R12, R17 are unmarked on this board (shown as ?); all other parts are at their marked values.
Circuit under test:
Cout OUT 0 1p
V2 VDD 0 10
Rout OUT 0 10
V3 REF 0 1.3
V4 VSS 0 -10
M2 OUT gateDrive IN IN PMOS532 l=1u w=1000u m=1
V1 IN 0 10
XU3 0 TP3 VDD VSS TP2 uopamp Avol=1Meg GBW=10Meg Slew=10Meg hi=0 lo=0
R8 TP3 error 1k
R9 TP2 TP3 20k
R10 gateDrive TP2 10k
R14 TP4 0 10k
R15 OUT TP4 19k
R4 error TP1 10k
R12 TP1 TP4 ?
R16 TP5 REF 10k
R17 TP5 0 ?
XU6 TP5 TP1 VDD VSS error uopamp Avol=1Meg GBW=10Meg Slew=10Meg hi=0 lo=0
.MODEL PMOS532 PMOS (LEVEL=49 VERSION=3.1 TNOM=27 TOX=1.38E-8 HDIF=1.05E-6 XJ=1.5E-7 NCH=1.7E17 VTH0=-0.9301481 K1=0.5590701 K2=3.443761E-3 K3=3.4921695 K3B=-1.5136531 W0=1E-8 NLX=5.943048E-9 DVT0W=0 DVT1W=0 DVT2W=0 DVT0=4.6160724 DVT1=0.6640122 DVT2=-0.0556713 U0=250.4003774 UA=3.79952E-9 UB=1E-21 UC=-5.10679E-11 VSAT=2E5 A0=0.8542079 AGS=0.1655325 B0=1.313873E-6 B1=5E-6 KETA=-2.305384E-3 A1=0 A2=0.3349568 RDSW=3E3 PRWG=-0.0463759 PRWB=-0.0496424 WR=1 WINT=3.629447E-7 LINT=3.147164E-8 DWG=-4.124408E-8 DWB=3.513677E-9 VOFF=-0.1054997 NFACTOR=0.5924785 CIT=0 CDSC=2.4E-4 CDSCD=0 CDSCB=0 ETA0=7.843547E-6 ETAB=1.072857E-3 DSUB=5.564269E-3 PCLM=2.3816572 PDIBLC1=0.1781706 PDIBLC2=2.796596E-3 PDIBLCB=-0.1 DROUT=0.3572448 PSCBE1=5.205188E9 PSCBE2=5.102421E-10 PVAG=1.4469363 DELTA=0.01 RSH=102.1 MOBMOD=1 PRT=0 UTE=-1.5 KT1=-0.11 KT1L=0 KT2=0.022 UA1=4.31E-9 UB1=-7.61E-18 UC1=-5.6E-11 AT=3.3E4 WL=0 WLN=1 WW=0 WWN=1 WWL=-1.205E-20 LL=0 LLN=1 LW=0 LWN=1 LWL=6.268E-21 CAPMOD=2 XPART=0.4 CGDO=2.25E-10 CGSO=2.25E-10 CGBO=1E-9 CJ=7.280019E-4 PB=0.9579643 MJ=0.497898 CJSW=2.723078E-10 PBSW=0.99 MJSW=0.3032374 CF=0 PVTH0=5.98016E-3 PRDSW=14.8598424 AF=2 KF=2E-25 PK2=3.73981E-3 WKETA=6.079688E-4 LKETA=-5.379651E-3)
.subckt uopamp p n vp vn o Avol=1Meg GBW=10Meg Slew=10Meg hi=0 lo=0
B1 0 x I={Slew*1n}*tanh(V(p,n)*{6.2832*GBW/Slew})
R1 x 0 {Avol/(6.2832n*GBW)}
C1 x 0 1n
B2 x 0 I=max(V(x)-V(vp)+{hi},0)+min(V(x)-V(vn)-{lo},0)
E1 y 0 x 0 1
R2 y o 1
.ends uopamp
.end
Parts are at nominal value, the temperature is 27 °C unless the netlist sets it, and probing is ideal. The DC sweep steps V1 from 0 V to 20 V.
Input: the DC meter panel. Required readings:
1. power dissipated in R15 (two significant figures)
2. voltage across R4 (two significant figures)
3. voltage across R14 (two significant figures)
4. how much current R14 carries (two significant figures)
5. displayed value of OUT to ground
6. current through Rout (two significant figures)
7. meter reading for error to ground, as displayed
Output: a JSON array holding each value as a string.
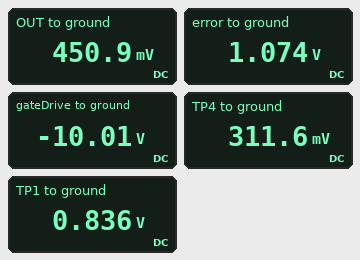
["1.0 µW", "240 mV", "310 mV", "31 µA", "450.9 mV", "45 mA", "1.074 V"]
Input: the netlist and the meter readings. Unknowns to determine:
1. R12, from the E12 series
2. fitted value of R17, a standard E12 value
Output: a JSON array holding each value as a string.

["22 kΩ", "18 kΩ"]
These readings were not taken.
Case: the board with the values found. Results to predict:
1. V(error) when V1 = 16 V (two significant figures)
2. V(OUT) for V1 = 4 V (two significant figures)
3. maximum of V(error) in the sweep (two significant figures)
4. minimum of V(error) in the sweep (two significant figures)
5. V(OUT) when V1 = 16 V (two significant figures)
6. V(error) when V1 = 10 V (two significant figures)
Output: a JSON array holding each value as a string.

["1.0 V", "180 mV", "1.1 V", "1.0 V", "720 mV", "1.1 V"]
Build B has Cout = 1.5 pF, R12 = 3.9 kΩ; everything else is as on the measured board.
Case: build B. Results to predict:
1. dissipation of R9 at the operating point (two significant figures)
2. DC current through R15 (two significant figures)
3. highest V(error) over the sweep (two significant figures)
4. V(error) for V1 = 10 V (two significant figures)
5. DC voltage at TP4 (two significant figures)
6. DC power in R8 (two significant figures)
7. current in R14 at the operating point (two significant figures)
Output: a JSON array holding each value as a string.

["6.0 mW", "6.9 µA", "1.6 V", "1.5 V", "580 mV", "300 µW", "58 µA"]
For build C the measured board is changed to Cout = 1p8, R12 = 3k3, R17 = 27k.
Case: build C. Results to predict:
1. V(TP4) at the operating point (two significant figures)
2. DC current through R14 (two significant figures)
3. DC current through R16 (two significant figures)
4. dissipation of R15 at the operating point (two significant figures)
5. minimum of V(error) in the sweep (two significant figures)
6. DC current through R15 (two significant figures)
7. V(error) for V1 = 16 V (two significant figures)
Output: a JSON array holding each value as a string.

["680 mV", "68 µA", "35 µA", "2.8 µW", "1.6 V", "12 µA", "1.7 V"]
